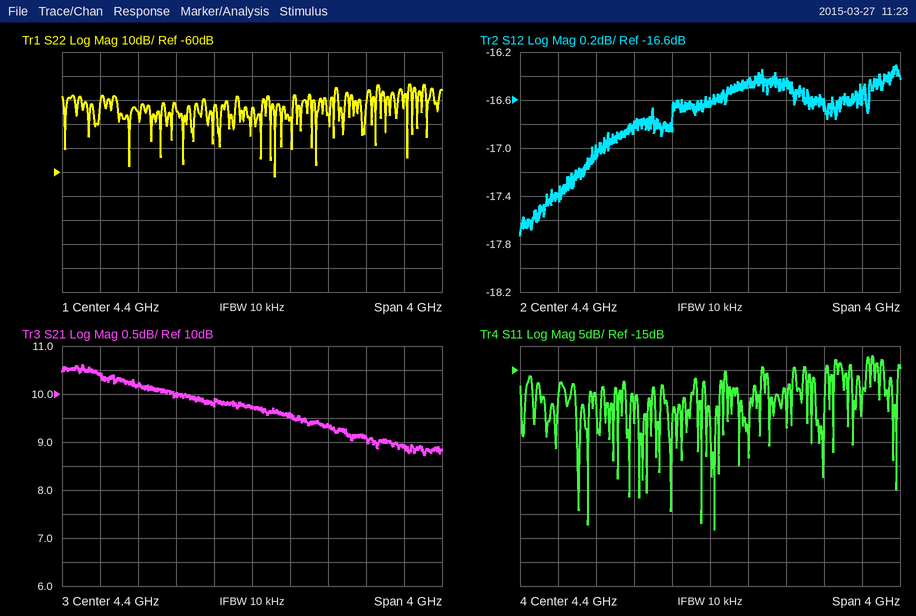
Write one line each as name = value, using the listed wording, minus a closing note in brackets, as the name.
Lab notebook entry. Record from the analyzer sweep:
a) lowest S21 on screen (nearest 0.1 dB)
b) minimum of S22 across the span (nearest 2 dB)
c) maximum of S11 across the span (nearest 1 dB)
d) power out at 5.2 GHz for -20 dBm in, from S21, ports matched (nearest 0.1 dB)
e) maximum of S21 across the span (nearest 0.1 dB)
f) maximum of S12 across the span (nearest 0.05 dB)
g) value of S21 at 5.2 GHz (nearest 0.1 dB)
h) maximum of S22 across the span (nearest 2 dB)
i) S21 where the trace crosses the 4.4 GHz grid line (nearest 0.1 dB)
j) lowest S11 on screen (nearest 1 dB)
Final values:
lowest S21 on screen = 8.7 dB
minimum of S22 across the span = -62 dB
maximum of S11 across the span = -12 dB
power out at 5.2 GHz for -20 dBm in, from S21, ports matched = -10.7 dBm
maximum of S21 across the span = 10.6 dB
maximum of S12 across the span = -16.30 dB
value of S21 at 5.2 GHz = 9.3 dB
maximum of S22 across the span = -24 dB
S21 where the trace crosses the 4.4 GHz grid line = 9.7 dB
lowest S11 on screen = -48 dB
